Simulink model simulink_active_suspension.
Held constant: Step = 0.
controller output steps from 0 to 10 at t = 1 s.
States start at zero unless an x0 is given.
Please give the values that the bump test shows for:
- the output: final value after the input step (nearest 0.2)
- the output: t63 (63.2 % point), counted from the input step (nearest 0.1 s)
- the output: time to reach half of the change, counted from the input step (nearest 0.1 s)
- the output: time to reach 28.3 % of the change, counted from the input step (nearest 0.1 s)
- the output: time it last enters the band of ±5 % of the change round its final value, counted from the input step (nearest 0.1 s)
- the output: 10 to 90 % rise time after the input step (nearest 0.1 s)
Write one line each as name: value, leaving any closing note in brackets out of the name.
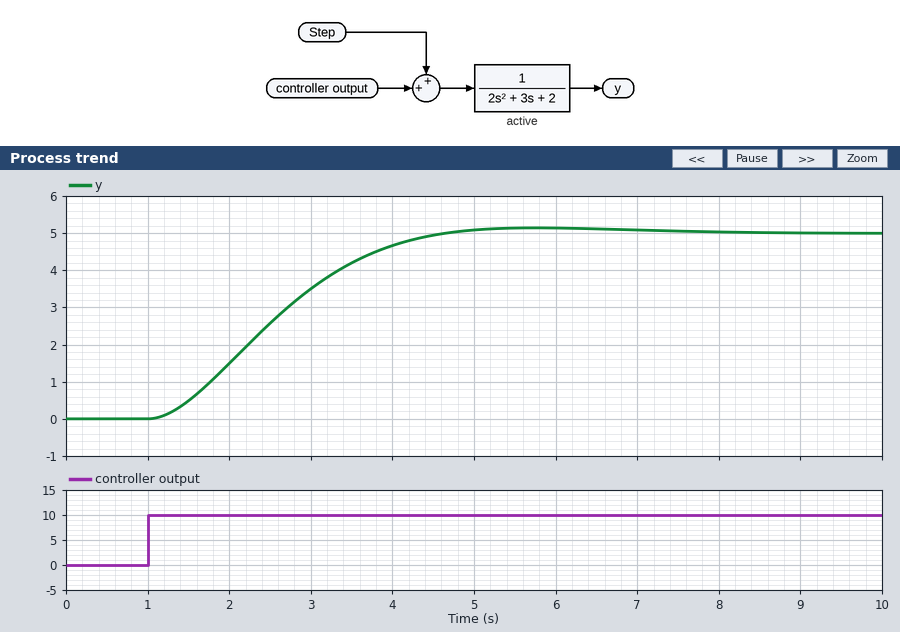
the output: final value after the input step: 5.0
the output: t63 (63.2 % point), counted from the input step: 1.8 s
the output: time to reach half of the change, counted from the input step: 1.5 s
the output: time to reach 28.3 % of the change, counted from the input step: 1.0 s
the output: time it last enters the band of ±5 % of the change round its final value, counted from the input step: 3.1 s
the output: 10 to 90 % rise time after the input step: 2.3 s
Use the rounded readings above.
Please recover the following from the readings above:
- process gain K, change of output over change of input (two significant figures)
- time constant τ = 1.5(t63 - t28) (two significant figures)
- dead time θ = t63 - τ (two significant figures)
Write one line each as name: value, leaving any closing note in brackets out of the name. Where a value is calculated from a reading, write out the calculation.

process gain K, change of output over change of input: (5 - 0) / 10 = 0.50
time constant τ = 1.5(t63 - t28): 1.5 × (1.8 - 1) = 1.2 s
dead time θ = t63 - τ: 1.8 - 1.2 = 0.60 s
